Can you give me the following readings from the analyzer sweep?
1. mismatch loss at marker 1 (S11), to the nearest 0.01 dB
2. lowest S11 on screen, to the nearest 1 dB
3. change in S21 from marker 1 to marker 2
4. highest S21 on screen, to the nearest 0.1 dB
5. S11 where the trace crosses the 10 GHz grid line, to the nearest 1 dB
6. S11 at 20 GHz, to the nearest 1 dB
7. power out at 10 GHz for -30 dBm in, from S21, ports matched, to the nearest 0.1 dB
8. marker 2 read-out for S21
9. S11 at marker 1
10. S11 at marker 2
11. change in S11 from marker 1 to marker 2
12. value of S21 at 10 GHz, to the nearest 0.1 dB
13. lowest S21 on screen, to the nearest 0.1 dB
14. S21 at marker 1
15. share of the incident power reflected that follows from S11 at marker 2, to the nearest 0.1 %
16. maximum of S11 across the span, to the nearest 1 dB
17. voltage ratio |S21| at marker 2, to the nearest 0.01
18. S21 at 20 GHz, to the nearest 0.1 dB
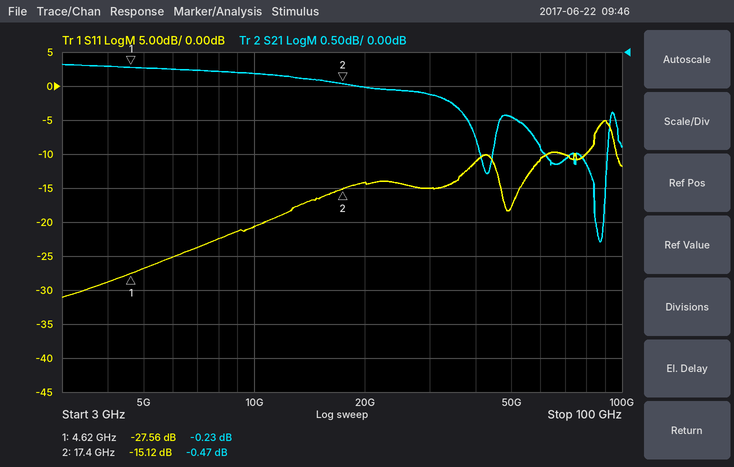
0.01 dB
-31 dB
-0.24 dB
-0.2 dB
-21 dB
-14 dB
-30.3 dBm
-0.47 dB
-27.56 dB
-15.12 dB
12.44 dB
-0.3 dB
-2.8 dB
-0.23 dB
3.1 %
-5 dB
0.95
-0.5 dB
